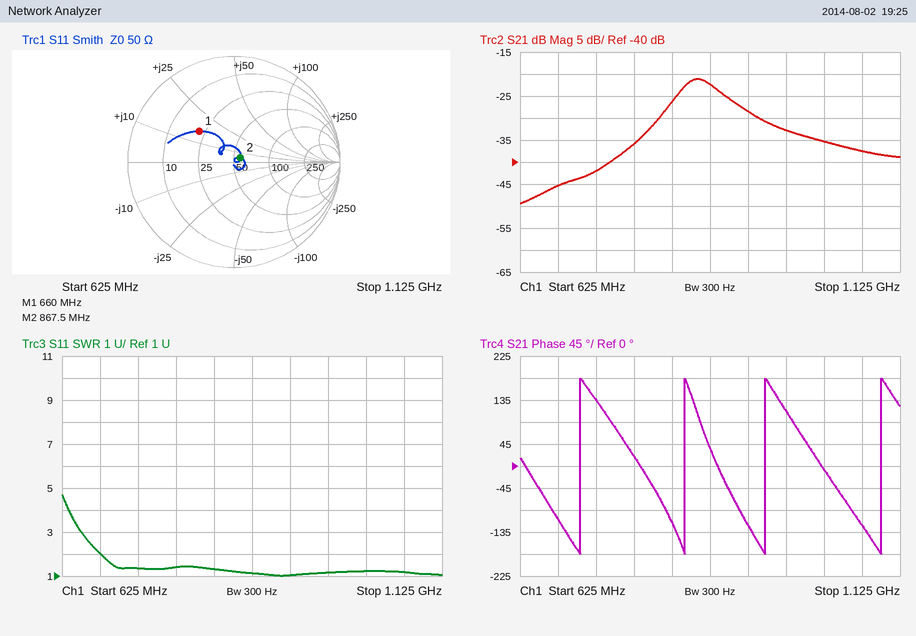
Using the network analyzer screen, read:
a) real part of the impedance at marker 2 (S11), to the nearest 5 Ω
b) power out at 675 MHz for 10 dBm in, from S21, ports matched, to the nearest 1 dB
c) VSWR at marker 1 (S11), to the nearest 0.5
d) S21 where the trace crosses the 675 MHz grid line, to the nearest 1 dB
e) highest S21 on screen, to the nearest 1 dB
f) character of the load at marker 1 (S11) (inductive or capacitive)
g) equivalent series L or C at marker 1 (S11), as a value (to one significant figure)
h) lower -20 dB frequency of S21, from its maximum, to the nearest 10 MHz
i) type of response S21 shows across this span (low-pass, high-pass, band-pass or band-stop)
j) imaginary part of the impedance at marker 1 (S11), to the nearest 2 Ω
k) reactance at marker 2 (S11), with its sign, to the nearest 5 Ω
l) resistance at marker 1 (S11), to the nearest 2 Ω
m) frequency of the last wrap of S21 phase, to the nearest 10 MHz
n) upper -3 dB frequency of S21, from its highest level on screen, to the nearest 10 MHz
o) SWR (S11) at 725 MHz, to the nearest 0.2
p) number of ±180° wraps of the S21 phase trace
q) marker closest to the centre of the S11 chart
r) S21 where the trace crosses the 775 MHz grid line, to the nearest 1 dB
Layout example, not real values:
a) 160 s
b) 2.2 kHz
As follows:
a) 55 Ω
b) -35 dBm
c) 2.5
d) -45 dB
e) -21 dB
f) inductive
g) 4 nH
h) 730 MHz
i) band-pass
j) +16 Ω
k) +5 Ω
l) 22 Ω
m) 1.10 GHz
n) 890 MHz
o) 1.4
p) 4
q) marker 2
r) -36 dB
